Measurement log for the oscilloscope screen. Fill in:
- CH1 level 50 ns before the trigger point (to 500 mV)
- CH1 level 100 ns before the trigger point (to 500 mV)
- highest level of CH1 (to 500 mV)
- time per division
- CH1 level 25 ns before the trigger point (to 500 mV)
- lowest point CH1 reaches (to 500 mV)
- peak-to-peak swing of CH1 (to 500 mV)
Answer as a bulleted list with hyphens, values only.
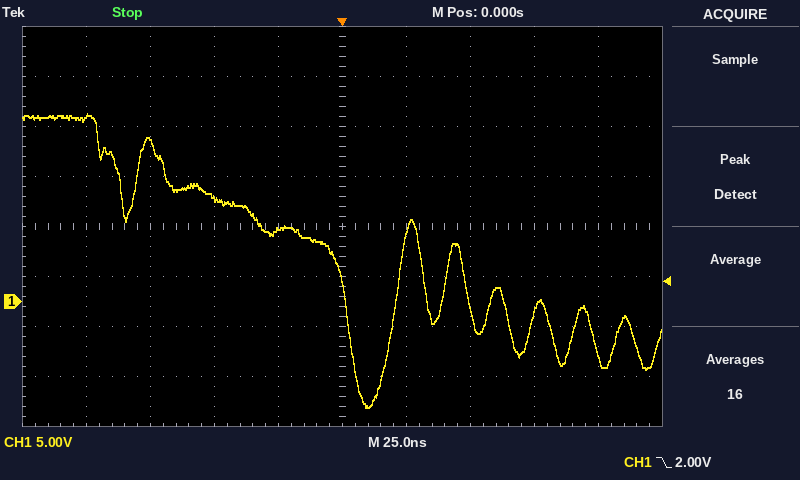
- 10.5 V
- 18.5 V
- 19.0 V
- 25 ns
- 7.0 V
- -10.5 V
- 29.5 V
